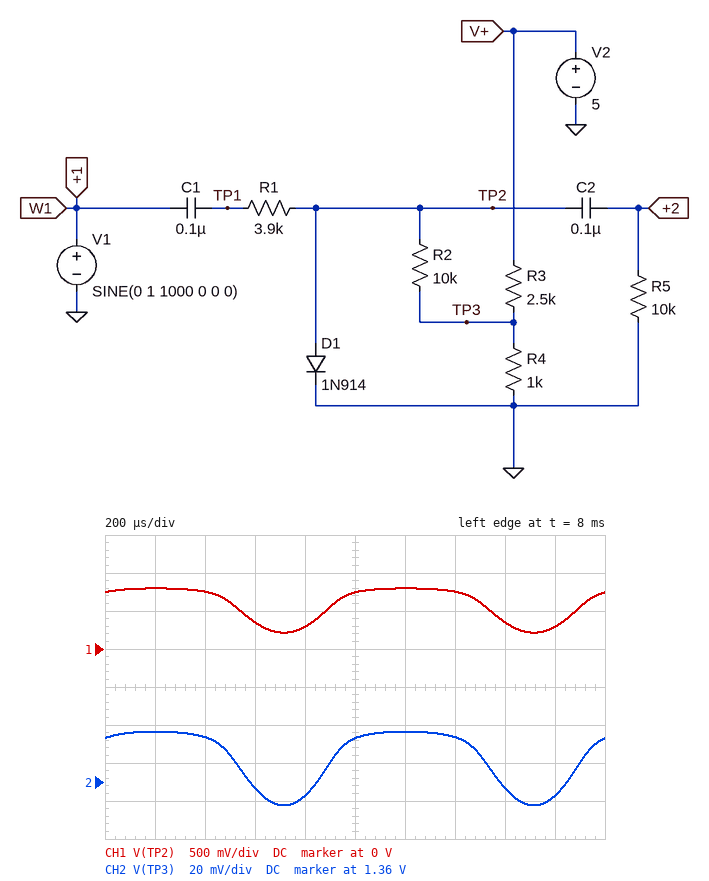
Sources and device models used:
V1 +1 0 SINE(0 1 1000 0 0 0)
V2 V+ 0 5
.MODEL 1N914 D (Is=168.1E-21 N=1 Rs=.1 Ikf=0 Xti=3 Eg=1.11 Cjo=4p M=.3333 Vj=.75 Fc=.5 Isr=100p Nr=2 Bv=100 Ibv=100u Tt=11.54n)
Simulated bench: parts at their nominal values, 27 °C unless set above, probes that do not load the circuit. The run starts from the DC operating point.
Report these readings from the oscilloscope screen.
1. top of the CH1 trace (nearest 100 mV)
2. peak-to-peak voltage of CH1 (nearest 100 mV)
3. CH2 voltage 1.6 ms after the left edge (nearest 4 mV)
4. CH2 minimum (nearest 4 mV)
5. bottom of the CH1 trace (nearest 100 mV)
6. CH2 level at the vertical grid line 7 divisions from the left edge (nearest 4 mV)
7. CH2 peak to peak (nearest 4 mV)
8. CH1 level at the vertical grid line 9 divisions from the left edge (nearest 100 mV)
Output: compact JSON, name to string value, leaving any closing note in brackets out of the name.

{"top of the CH1 trace": "800 mV", "peak-to-peak voltage of CH1": "600 mV", "CH2 voltage 1.6 ms after the left edge": "1.356 V", "CH2 minimum": "1.348 V", "bottom of the CH1 trace": "200 mV", "CH2 level at the vertical grid line 7 divisions from the left edge": "1.384 V", "CH2 peak to peak": "40 mV", "CH1 level at the vertical grid line 9 divisions from the left edge": "300 mV"}
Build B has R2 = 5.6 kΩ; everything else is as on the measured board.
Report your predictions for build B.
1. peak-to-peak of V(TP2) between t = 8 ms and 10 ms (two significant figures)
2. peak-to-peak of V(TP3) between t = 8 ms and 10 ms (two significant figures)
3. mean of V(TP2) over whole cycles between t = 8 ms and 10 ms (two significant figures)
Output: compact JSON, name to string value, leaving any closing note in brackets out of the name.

{"peak-to-peak of V(TP2) between t = 8 ms and 10 ms": "370 mV", "peak-to-peak of V(TP3) between t = 8 ms and 10 ms": "42 mV", "mean of V(TP2) over whole cycles between t = 8 ms and 10 ms": "690 mV"}
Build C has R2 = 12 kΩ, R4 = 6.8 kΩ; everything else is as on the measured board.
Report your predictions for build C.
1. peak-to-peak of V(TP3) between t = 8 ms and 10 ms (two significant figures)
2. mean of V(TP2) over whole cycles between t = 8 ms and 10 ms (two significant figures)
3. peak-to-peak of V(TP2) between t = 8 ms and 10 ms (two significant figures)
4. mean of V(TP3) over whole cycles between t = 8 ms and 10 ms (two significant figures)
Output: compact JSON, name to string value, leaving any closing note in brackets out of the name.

{"peak-to-peak of V(TP3) between t = 8 ms and 10 ms": "22 mV", "mean of V(TP2) over whole cycles between t = 8 ms and 10 ms": "770 mV", "peak-to-peak of V(TP2) between t = 8 ms and 10 ms": "170 mV", "mean of V(TP3) over whole cycles between t = 8 ms and 10 ms": "3.3 V"}
